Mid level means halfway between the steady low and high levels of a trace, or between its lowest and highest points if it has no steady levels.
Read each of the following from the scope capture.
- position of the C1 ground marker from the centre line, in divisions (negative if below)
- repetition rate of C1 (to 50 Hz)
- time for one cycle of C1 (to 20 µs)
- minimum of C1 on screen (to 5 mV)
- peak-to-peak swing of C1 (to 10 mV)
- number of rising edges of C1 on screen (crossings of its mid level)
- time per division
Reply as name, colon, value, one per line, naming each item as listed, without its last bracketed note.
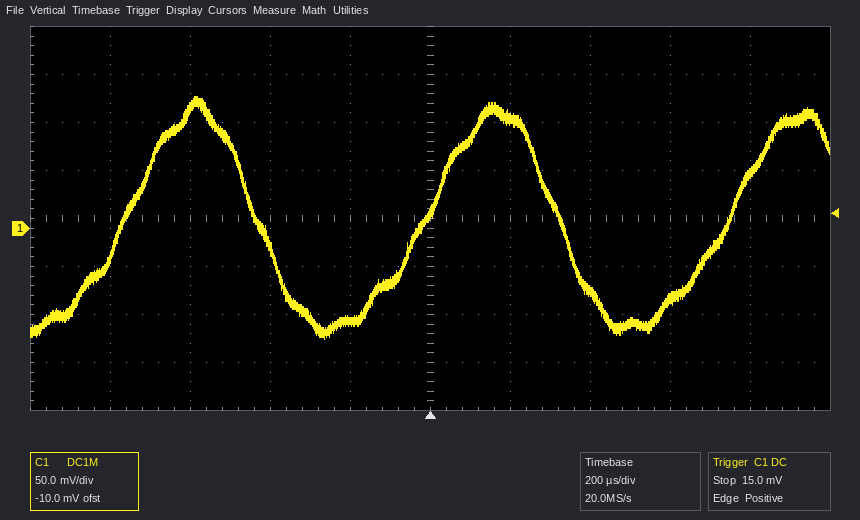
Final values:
position of the C1 ground marker from the centre line, in divisions: -0.2 div
repetition rate of C1: 1.30 kHz
time for one cycle of C1: 760 µs
minimum of C1 on screen: -115 mV
peak-to-peak swing of C1: 250 mV
number of rising edges of C1 on screen: 3
time per division: 200 µs
